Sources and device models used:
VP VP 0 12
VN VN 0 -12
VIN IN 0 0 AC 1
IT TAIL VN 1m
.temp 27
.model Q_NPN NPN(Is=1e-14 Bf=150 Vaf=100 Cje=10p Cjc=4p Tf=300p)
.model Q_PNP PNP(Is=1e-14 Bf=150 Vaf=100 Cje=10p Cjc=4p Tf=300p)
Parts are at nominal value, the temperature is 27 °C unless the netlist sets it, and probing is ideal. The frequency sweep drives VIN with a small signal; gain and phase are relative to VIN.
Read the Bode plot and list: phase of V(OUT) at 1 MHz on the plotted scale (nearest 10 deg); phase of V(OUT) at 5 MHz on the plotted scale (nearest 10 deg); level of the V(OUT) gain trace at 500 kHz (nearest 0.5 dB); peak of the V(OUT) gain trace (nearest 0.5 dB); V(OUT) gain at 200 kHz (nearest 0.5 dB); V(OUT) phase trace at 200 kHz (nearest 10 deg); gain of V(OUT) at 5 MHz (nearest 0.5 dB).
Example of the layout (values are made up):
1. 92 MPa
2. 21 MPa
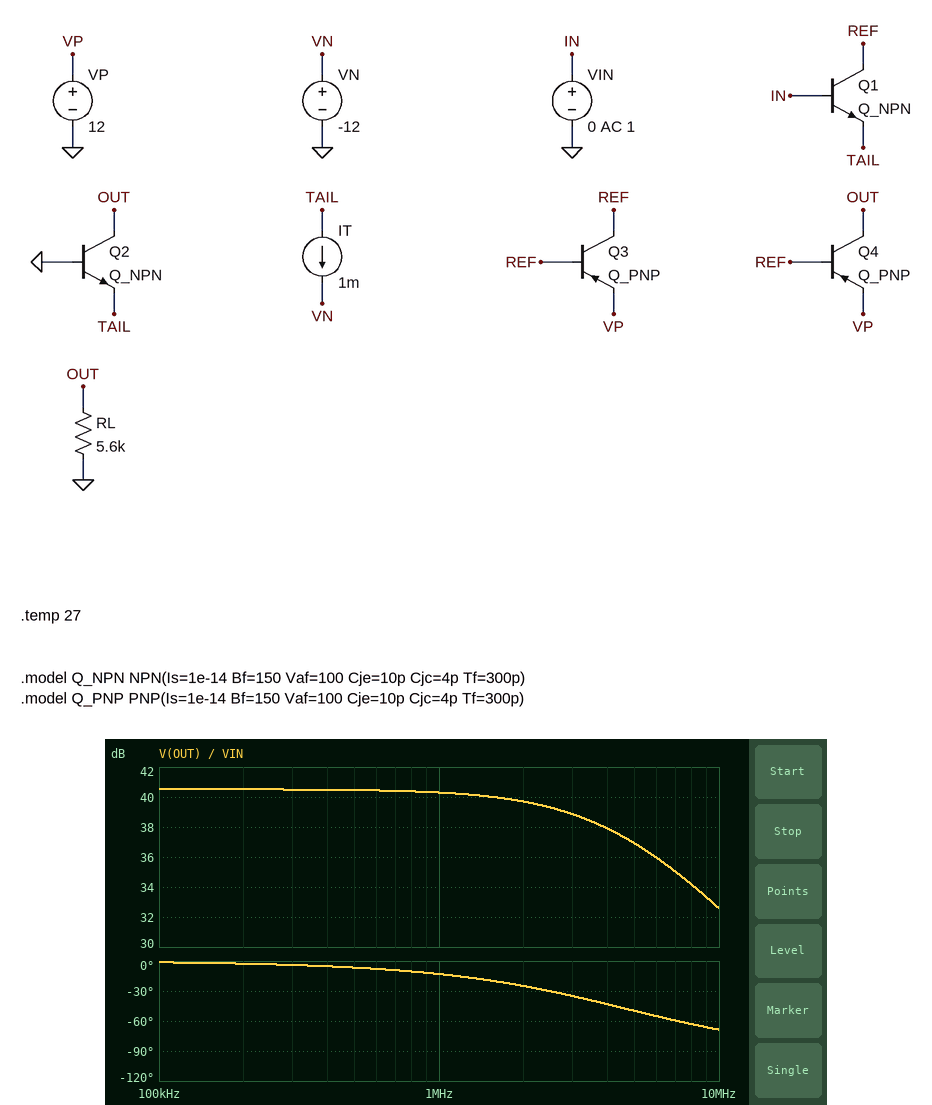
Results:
1. -10 deg
2. -50 deg
3. 40.5 dB
4. 40.5 dB
5. 40.5 dB
6. 0 deg
7. 37.0 dB
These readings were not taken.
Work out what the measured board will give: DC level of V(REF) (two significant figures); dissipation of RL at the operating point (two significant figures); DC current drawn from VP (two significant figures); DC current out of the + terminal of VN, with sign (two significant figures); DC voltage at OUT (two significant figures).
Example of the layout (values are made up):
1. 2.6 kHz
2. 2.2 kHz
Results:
1. 11 V
2. 55 µW
3. 1.1 mA
4. -1.0 mA
5. 560 mV
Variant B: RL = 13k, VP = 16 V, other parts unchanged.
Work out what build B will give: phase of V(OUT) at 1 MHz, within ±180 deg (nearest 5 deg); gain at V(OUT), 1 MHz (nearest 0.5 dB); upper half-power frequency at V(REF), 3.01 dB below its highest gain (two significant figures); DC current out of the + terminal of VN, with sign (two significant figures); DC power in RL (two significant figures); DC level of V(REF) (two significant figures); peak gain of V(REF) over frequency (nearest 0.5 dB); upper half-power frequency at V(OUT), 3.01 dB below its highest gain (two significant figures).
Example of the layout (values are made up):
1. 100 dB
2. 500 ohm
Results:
1. -25 deg
2. 46.5 dB
3. 3.2 MHz
4. -1.0 mA
5. 210 µW
6. 15 V
7. -7.0 dB
8. 2.3 MHz
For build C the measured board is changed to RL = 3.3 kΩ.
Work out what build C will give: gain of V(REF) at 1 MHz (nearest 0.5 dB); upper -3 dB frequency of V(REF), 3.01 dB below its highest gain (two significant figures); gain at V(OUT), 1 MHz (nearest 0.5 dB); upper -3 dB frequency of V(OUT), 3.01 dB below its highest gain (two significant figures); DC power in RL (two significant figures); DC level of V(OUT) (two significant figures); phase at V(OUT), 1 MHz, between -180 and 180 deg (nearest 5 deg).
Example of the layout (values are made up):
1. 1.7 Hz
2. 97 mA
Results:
1. -6.5 dB
2. 9.9 MHz
3. 36.0 dB
4. 7.0 MHz
5. 34 µW
6. 340 mV
7. -10 deg
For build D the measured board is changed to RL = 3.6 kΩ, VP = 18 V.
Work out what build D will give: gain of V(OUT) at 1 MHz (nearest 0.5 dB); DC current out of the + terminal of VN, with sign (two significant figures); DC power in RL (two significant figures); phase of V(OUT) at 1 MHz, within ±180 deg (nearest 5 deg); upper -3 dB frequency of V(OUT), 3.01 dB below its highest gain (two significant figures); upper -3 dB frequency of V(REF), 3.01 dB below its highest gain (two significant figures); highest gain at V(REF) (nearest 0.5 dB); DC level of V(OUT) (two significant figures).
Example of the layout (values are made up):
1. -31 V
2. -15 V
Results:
1. 37.0 dB
2. -1.0 mA
3. 90 µW
4. -10 deg
5. 7.0 MHz
6. 10 MHz
7. -7.0 dB
8. 570 mV
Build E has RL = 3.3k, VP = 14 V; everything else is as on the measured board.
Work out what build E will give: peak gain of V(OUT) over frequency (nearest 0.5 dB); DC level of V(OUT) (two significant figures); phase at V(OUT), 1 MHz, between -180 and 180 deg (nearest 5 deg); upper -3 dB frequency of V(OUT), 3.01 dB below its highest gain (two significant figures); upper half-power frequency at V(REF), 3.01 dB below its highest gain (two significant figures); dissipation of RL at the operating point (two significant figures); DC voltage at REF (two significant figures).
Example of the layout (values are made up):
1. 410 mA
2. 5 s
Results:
1. 36.0 dB
2. 400 mV
3. -10 deg
4. 7.2 MHz
5. 10 MHz
6. 48 µW
7. 13 V
